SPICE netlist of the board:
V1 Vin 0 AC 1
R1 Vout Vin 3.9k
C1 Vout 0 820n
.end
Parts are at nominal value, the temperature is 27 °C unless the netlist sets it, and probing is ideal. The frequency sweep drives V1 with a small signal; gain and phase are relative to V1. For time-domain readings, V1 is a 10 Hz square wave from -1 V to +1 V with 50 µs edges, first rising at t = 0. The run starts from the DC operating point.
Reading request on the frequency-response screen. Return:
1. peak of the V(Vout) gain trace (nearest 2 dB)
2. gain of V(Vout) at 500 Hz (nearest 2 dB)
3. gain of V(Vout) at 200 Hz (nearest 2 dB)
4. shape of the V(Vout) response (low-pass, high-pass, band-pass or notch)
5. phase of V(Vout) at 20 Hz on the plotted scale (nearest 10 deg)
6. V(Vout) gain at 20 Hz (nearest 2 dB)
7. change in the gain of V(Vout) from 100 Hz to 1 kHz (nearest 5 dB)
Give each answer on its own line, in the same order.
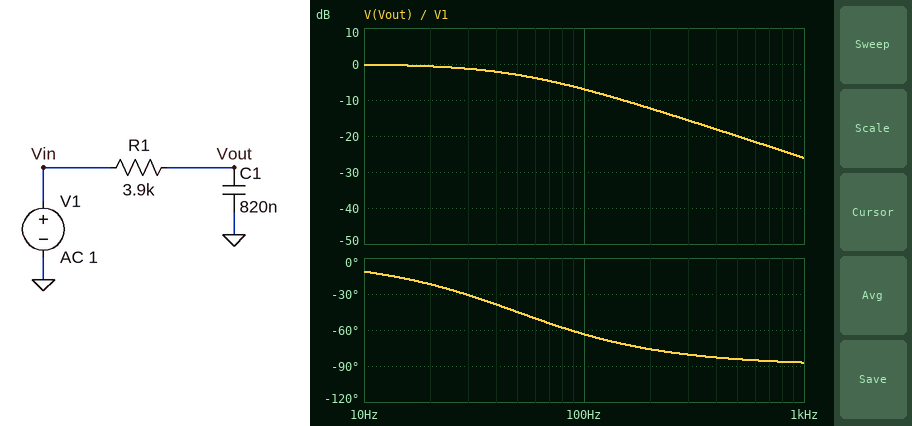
0 dB
-20 dB
-12 dB
low-pass
-20 deg
0 dB
-20 dB
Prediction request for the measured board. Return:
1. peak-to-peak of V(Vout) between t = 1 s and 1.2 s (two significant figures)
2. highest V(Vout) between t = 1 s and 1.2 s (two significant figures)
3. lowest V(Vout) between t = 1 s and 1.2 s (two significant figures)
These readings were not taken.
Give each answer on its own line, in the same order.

2.0 V
1.0 V
-1.0 V
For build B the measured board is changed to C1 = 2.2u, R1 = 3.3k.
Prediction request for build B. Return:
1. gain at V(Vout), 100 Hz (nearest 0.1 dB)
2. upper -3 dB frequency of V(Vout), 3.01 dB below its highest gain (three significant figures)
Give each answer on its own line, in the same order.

-13.4 dB
21.9 Hz
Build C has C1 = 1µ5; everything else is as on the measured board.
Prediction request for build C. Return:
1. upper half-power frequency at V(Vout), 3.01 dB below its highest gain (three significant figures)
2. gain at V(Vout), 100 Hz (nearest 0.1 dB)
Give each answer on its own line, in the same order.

27.2 Hz
-11.6 dB
